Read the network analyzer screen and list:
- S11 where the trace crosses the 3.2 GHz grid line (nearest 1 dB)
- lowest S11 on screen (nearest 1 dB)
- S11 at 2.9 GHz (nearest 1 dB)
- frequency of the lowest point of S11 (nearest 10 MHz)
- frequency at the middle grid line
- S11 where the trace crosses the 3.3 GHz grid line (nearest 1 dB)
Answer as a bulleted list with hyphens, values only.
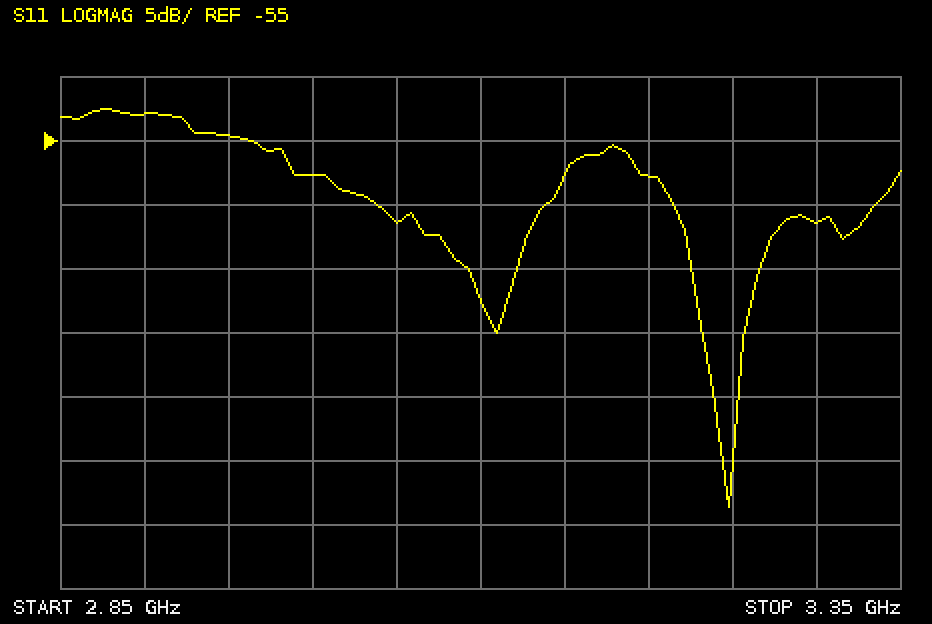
- -58 dB
- -84 dB
- -53 dB
- 3.25 GHz
- 3.1 GHz
- -61 dB
